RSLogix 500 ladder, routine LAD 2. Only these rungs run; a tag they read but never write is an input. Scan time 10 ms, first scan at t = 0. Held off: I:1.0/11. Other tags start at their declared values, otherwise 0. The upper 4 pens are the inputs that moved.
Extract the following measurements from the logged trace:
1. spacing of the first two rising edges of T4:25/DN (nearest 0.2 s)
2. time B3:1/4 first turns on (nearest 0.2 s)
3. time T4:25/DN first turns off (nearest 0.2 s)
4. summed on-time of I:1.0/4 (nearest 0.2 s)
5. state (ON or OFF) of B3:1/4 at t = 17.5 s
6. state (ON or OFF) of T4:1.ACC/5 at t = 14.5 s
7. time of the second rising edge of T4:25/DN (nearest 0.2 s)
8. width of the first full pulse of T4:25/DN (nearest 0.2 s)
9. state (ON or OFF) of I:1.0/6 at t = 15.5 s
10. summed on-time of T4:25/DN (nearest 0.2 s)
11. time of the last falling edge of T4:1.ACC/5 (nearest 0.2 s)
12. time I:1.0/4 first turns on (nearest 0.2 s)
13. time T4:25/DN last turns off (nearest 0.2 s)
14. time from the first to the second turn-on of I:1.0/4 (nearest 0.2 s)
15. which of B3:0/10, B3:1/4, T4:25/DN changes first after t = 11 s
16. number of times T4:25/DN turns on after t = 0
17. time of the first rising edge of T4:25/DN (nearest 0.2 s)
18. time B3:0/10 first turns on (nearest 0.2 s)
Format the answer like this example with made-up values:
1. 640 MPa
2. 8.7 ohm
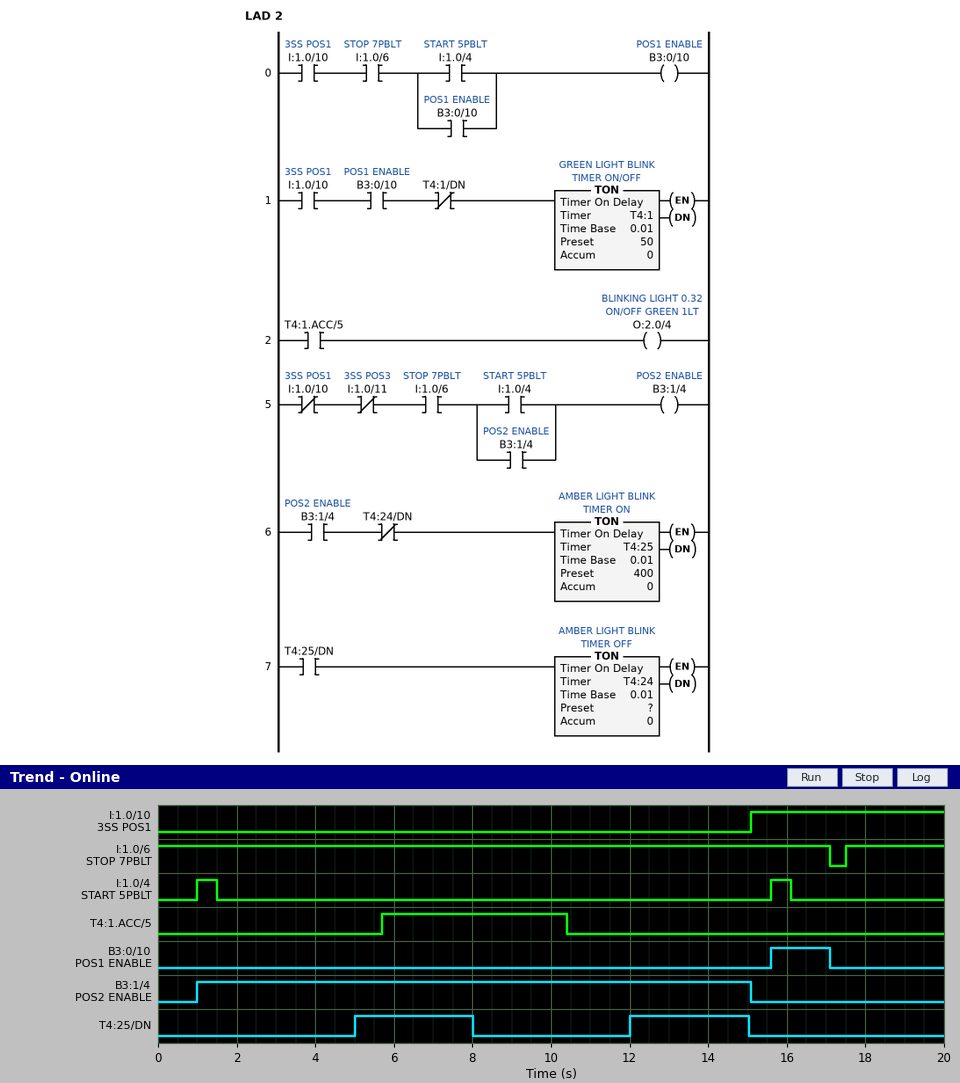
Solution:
1. 7.0 s
2. 1.0 s
3. 8.0 s
4. 1.0 s
5. OFF
6. OFF
7. 12.0 s
8. 3.0 s
9. ON
10. 6.0 s
11. 10.4 s
12. 1.0 s
13. 15.0 s
14. 14.6 s
15. T4:25/DN
16. 2
17. 5.0 s
18. 15.6 s
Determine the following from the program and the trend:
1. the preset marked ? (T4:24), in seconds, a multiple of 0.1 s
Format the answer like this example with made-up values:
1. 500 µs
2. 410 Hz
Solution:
1. 3.0 s
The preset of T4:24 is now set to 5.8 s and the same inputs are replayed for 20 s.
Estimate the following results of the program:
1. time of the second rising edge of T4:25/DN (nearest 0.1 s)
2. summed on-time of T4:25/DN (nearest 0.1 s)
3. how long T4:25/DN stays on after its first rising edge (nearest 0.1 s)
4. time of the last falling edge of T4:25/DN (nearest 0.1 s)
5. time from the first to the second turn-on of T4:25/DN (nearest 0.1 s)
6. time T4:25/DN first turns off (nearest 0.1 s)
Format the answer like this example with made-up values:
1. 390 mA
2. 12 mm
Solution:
1. 14.8 s
2. 6.1 s
3. 5.8 s
4. 15.1 s
5. 9.8 s
6. 10.8 s
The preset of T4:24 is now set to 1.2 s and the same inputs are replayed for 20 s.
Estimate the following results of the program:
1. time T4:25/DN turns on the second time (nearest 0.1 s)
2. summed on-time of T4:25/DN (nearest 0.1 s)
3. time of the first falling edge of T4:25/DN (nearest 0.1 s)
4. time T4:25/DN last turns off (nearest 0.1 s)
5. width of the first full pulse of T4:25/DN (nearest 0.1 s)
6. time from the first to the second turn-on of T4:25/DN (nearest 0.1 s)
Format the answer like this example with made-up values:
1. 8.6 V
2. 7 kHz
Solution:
1. 10.2 s
2. 2.4 s
3. 6.2 s
4. 11.4 s
5. 1.2 s
6. 5.2 s
